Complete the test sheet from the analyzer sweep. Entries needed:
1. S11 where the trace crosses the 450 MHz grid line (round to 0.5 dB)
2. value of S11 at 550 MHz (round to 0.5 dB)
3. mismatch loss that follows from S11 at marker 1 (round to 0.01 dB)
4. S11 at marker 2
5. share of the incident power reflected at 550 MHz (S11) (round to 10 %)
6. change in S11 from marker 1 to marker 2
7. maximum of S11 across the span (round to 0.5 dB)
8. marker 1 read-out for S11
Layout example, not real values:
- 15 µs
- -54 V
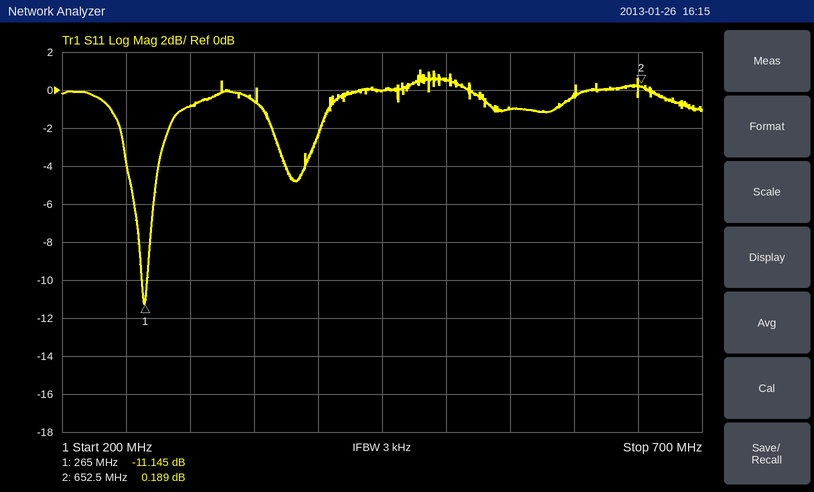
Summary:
- 0.0 dB
- -1.0 dB
- 0.35 dB
- 0.189 dB
- 80 %
- 11.334 dB
- 1.0 dB
- -11.145 dB
